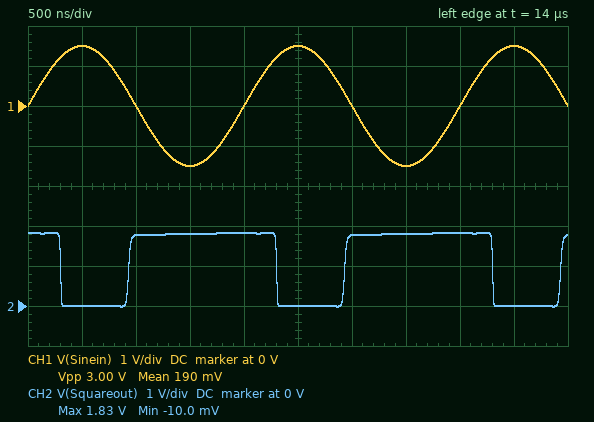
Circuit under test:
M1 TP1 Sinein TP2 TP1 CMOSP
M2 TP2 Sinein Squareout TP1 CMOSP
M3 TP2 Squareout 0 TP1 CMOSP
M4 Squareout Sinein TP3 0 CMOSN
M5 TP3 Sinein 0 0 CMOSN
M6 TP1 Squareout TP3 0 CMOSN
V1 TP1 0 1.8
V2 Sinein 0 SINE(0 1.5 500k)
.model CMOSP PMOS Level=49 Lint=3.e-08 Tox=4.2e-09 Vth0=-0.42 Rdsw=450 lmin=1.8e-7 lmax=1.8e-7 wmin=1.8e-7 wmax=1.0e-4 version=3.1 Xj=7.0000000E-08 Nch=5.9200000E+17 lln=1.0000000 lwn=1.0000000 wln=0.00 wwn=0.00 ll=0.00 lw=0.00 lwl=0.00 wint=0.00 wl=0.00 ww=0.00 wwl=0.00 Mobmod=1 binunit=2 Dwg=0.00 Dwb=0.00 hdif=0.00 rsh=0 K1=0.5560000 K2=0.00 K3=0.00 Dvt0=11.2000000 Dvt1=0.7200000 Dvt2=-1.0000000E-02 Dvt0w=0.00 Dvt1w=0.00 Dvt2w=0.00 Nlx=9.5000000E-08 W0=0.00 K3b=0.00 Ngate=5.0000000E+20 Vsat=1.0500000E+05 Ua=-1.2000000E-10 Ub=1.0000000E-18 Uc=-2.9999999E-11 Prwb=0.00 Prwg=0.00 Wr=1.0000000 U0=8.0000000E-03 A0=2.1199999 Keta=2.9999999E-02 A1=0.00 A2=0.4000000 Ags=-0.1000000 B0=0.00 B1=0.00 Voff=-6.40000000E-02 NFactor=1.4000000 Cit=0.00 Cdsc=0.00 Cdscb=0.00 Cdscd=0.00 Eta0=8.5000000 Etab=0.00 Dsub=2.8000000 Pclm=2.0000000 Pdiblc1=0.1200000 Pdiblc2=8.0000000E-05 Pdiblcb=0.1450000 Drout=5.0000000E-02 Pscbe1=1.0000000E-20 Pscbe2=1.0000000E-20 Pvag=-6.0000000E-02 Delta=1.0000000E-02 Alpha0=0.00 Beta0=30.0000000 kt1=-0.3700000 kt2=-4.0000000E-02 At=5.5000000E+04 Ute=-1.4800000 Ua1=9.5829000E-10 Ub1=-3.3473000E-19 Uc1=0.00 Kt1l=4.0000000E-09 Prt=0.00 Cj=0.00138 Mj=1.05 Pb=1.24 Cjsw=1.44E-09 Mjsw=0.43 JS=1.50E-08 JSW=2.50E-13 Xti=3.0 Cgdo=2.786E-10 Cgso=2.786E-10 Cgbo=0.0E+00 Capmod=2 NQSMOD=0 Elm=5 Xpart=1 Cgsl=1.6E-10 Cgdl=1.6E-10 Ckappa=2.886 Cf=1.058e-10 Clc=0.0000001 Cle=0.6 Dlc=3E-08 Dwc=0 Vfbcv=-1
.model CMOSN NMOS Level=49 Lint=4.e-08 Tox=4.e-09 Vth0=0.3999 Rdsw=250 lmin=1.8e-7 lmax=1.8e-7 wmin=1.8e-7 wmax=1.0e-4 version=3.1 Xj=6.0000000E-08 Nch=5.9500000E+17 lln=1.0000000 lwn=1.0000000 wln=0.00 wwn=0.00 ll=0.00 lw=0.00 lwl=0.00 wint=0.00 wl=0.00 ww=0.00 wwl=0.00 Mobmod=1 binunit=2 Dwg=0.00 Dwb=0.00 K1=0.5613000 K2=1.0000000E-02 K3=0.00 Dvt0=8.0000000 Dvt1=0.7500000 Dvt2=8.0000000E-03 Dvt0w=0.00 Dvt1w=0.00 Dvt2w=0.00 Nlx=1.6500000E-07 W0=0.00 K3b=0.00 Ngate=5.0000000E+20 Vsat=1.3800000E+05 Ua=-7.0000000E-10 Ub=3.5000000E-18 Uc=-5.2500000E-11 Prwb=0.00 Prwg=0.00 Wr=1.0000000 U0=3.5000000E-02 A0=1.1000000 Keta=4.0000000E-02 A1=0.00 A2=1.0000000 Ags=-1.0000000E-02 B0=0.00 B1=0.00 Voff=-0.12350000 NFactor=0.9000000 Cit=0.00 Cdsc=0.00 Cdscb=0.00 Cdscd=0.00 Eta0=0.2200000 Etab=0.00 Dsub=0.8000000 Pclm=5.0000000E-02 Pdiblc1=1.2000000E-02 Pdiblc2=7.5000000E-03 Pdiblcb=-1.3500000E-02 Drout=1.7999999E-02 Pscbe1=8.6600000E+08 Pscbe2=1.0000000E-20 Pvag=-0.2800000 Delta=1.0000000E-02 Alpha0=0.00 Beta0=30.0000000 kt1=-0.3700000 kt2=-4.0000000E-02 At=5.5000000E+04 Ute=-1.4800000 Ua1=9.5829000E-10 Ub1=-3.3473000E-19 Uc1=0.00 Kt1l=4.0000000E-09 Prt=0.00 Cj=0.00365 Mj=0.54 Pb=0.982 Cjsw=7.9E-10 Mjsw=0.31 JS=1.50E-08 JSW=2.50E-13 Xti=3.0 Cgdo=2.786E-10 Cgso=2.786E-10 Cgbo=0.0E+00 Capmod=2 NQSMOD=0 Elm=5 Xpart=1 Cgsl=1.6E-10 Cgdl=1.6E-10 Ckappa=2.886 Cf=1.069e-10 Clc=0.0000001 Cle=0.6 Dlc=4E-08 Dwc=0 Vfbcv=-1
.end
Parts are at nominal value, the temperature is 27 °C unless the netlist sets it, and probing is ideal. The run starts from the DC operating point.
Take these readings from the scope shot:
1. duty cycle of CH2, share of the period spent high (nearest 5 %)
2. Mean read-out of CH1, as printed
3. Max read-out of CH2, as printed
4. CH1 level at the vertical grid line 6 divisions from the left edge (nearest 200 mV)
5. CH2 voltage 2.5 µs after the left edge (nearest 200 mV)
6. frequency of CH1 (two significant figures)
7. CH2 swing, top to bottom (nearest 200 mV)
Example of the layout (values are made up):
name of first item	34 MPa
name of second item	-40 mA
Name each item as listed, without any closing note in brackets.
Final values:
duty cycle of CH2, share of the period spent high	70 %
Mean read-out of CH1, as printed	190 mV
Max read-out of CH2, as printed	1.83 V
CH1 level at the vertical grid line 6 divisions from the left edge	0 V
CH2 voltage 2.5 µs after the left edge	0 V
frequency of CH1	500 kHz
CH2 swing, top to bottom	1.8 V
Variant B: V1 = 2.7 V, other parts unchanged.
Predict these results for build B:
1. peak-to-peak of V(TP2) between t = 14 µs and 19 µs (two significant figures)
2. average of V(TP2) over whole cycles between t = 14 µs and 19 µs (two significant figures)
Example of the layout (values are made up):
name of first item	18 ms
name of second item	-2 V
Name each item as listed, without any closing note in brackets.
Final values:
peak-to-peak of V(TP2) between t = 14 µs and 19 µs	31 mV
average of V(TP2) over whole cycles between t = 14 µs and 19 µs	2.7 V
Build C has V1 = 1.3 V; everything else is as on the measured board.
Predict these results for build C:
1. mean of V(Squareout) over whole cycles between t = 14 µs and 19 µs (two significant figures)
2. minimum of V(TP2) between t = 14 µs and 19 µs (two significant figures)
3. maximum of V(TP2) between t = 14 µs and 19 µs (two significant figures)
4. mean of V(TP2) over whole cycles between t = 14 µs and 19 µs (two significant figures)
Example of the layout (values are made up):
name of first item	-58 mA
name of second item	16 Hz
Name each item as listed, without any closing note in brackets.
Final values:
mean of V(Squareout) over whole cycles between t = 14 µs and 19 µs	820 mV
minimum of V(TP2) between t = 14 µs and 19 µs	510 mV
maximum of V(TP2) between t = 14 µs and 19 µs	1.4 V
mean of V(TP2) over whole cycles between t = 14 µs and 19 µs	1.1 V
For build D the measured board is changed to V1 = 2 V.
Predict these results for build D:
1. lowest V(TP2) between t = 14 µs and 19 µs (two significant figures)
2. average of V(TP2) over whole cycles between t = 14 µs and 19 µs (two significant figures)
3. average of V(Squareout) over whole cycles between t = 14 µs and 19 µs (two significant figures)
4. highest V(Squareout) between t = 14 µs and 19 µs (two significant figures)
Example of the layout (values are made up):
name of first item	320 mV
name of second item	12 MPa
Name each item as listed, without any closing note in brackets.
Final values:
lowest V(TP2) between t = 14 µs and 19 µs	780 mV
average of V(TP2) over whole cycles between t = 14 µs and 19 µs	1.7 V
average of V(Squareout) over whole cycles between t = 14 µs and 19 µs	1.4 V
highest V(Squareout) between t = 14 µs and 19 µs	2.0 V
